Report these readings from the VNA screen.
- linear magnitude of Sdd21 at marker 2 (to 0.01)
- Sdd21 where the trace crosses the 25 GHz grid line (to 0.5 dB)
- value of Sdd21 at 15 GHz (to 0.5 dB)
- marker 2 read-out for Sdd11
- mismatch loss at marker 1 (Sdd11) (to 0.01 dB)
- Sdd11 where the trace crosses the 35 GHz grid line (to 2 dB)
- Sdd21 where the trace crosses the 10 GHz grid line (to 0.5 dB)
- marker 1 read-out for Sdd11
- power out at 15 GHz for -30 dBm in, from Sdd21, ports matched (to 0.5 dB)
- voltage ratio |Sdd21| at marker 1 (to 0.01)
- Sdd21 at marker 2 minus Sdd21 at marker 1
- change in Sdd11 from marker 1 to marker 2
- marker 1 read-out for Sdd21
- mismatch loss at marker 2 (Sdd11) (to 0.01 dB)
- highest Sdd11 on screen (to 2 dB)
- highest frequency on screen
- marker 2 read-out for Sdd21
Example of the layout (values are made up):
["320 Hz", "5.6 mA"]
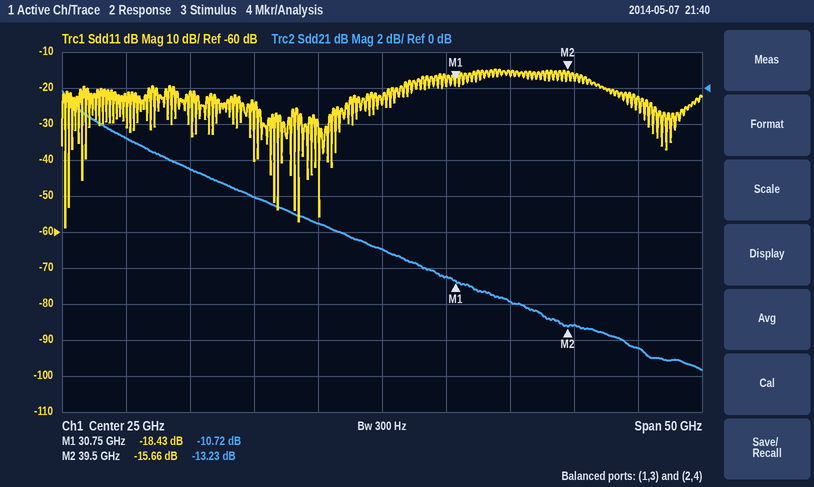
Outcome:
["0.22", "-9.0 dB", "-6.0 dB", "-15.66 dB", "0.06 dB", "-16 dB", "-4.5 dB", "-18.43 dB", "-36.0 dBm", "0.29", "-2.51 dB", "2.77 dB", "-10.72 dB", "0.12 dB", "-14 dB", "50 GHz", "-13.23 dB"]
